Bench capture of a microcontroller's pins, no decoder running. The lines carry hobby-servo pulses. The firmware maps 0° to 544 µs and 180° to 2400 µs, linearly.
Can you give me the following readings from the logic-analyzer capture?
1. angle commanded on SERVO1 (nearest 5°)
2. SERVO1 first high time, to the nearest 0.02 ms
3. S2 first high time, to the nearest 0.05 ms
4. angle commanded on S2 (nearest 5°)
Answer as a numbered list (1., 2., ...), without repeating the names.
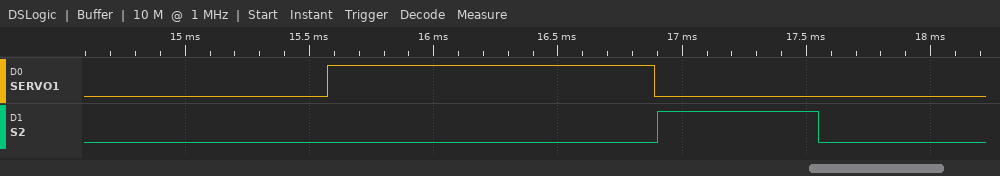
1. 75°
2. 1.32 ms
3. 0.65 ms
4. 10°
